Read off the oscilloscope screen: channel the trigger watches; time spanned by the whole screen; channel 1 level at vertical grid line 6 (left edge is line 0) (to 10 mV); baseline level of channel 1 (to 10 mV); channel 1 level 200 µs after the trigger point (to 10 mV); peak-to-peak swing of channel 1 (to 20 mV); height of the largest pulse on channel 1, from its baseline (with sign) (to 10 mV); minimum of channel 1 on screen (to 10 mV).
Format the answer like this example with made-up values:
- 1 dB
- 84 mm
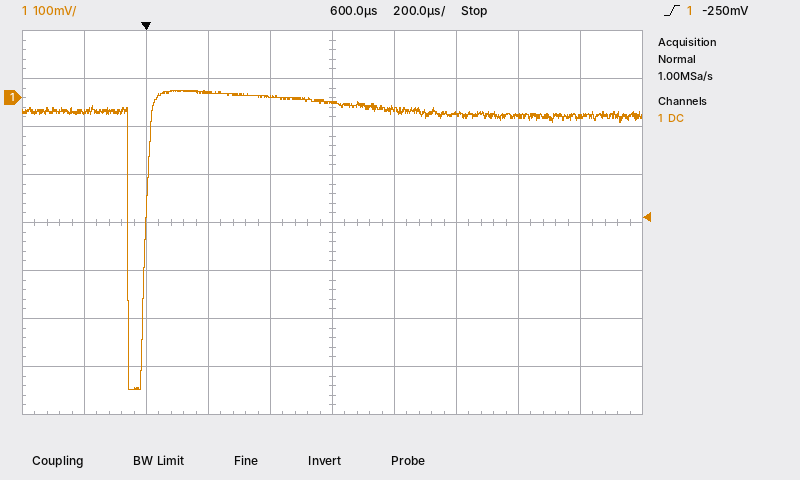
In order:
- channel 1
- 2 ms
- -20 mV
- -30 mV
- 10 mV
- 620 mV
- -580 mV
- -610 mV
